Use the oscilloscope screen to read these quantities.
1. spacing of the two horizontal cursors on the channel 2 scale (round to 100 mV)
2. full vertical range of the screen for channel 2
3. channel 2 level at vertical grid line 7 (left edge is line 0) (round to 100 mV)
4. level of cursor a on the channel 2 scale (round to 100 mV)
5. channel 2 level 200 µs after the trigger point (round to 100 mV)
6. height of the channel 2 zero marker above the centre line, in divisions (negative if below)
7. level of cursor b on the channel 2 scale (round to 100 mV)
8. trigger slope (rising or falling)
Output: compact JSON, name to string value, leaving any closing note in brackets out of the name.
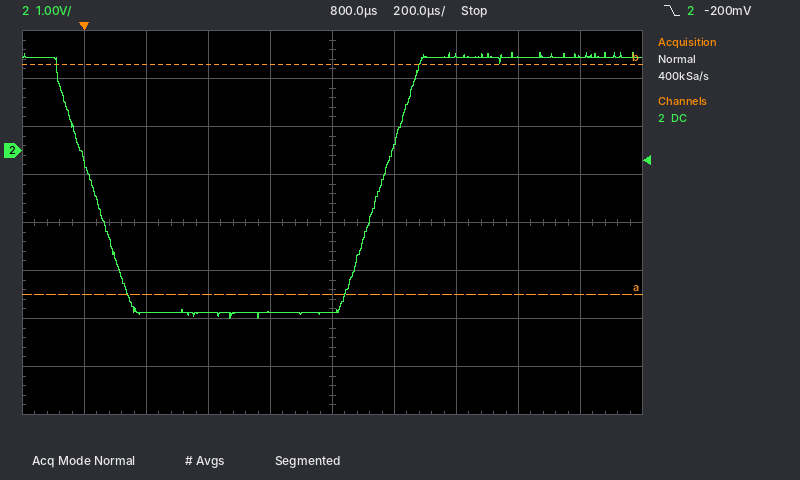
{"spacing of the two horizontal cursors on the channel 2 scale": "4.8 V", "full vertical range of the screen for channel 2": "8 V", "channel 2 level at vertical grid line 7 (left edge is line 0)": "2.0 V", "level of cursor a on the channel 2 scale": "-3.0 V", "channel 2 level 200 µs after the trigger point": "-3.4 V", "height of the channel 2 zero marker above the centre line, in divisions": "+1.5 div", "level of cursor b on the channel 2 scale": "1.8 V", "trigger slope": "falling"}
